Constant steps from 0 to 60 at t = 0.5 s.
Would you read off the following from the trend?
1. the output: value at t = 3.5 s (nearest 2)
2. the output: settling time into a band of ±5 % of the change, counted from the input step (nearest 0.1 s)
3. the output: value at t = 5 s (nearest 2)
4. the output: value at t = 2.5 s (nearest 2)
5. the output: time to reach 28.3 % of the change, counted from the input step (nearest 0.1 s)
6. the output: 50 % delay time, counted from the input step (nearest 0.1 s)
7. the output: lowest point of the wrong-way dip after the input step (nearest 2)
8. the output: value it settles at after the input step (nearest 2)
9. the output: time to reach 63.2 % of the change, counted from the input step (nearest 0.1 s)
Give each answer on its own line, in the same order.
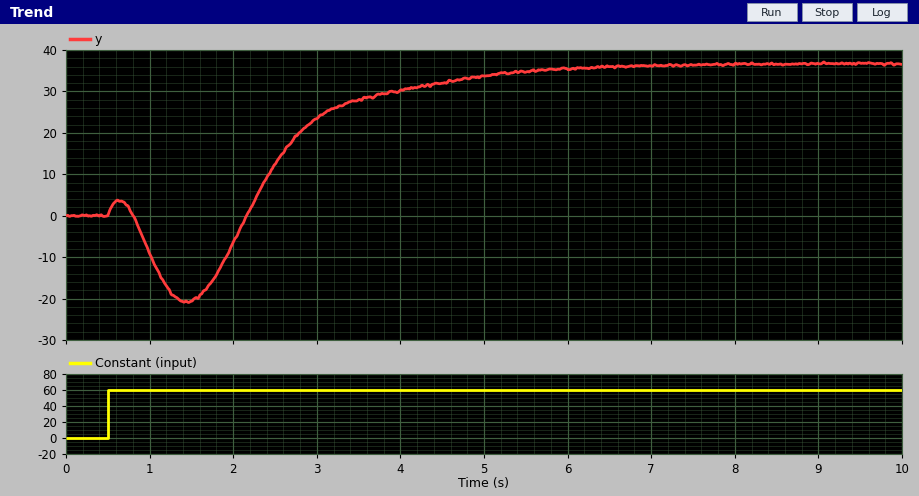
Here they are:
28
5.1 s
34
12
1.9 s
2.2 s
-20
36
2.5 s
